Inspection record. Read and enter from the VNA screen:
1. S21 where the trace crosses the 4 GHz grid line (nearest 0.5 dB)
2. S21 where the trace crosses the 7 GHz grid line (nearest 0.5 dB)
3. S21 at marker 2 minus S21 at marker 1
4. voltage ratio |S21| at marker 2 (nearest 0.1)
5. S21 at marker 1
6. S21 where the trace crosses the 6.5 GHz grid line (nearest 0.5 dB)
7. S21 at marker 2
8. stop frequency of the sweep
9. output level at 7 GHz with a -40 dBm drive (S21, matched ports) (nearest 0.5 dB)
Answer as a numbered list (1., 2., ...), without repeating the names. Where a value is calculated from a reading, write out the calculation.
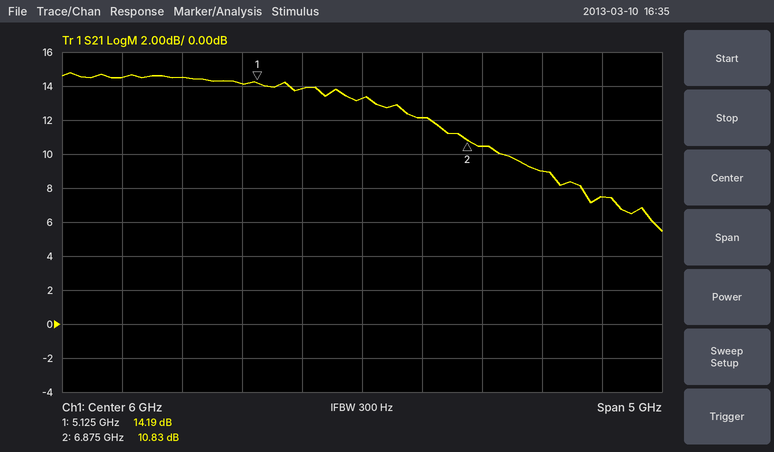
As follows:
1. 14.5 dB
2. 10.5 dB
3. 10.83 − (14.19) = -3.36 dB
4. 10^(10.83/20) ≈ 3.5
5. 14.19 dB
6. 12.0 dB
7. 10.83 dB
8. 8.5 GHz
9. -40 dBm + (10.5 dB) = -29.5 dBm
